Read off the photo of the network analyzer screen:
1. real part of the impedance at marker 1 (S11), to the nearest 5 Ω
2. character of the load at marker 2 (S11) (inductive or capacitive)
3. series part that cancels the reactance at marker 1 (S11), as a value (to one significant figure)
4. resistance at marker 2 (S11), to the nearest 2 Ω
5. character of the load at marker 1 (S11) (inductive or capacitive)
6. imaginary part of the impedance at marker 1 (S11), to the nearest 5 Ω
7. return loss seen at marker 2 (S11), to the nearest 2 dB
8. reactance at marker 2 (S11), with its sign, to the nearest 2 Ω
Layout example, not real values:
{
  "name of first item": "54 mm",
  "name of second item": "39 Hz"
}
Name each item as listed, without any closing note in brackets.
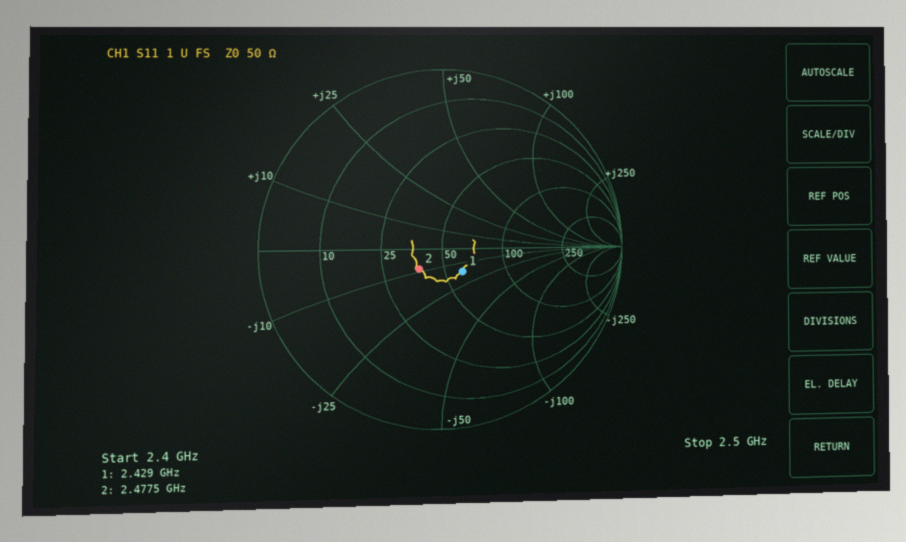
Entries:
{
  "real part of the impedance at marker 1 (S11), to the nearest 5 Ω": "60 Ω",
  "character of the load at marker 2 (S11)": "capacitive",
  "series part that cancels the reactance at marker 1 (S11), as a value": "1 nH",
  "resistance at marker 2 (S11), to the nearest 2 Ω": "38 Ω",
  "character of the load at marker 1 (S11)": "capacitive",
  "imaginary part of the impedance at marker 1 (S11), to the nearest 5 Ω": "-15 Ω",
  "return loss seen at marker 2 (S11), to the nearest 2 dB": "16 dB",
  "reactance at marker 2 (S11), with its sign, to the nearest 2 Ω": "-8 Ω"
}
